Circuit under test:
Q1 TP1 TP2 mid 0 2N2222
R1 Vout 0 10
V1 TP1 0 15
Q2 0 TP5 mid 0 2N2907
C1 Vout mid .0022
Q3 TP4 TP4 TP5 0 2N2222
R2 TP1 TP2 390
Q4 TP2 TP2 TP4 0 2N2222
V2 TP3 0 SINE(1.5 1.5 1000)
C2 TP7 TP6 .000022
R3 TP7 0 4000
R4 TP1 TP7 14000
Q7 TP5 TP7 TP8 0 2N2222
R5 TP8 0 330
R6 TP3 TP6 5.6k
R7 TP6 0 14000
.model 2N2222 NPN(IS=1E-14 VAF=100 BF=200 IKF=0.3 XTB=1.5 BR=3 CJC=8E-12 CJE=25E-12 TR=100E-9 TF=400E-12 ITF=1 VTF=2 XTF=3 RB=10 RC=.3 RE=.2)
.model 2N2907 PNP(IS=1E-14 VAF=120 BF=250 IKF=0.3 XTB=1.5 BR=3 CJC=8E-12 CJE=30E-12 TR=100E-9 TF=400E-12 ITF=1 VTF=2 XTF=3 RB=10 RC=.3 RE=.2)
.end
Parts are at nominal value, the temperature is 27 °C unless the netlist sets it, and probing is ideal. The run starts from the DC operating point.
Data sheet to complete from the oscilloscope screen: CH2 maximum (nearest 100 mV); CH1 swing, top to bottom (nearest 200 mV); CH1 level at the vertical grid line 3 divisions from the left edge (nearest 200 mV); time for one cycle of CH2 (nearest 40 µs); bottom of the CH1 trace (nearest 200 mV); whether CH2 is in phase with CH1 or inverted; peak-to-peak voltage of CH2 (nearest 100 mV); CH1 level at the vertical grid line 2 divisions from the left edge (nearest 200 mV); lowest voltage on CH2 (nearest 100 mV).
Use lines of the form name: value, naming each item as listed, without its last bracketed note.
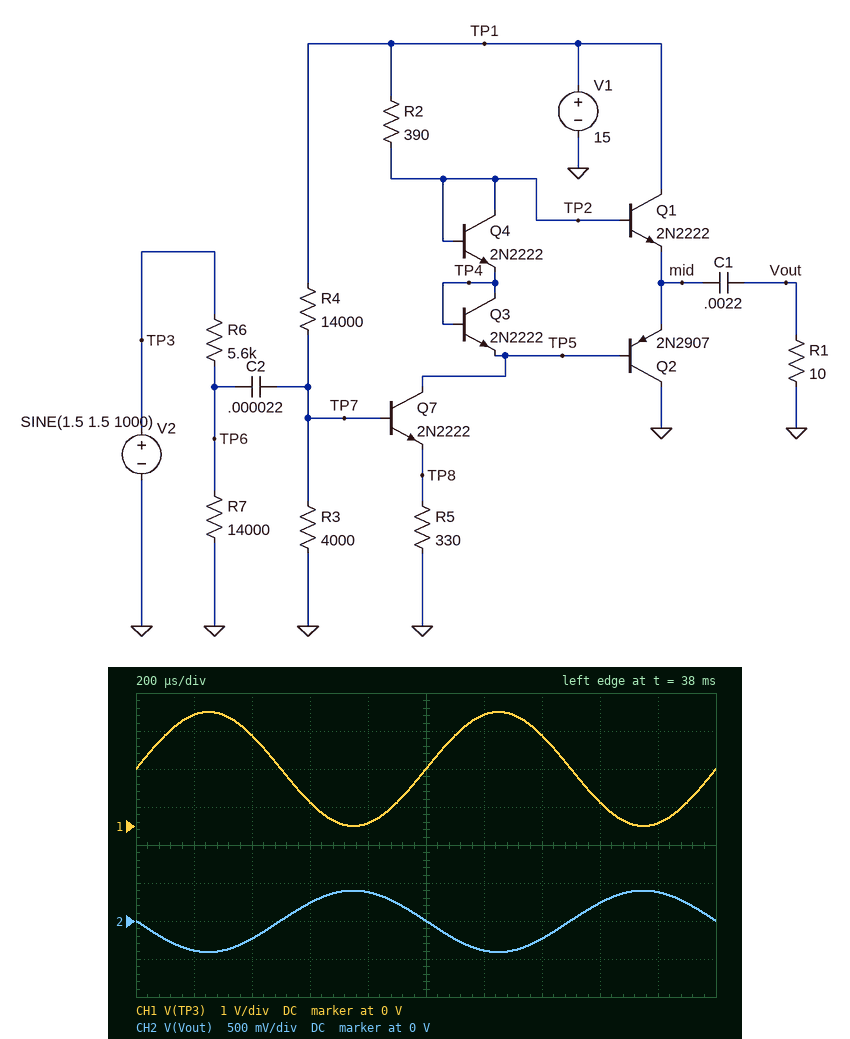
CH2 maximum: 400 mV
CH1 swing, top to bottom: 3.0 V
CH1 level at the vertical grid line 3 divisions from the left edge: 600 mV
time for one cycle of CH2: 1.00 ms
bottom of the CH1 trace: 0 V
whether CH2 is in phase with CH1 or inverted: inverted
peak-to-peak voltage of CH2: 800 mV
CH1 level at the vertical grid line 2 divisions from the left edge: 2.4 V
lowest voltage on CH2: -400 mV
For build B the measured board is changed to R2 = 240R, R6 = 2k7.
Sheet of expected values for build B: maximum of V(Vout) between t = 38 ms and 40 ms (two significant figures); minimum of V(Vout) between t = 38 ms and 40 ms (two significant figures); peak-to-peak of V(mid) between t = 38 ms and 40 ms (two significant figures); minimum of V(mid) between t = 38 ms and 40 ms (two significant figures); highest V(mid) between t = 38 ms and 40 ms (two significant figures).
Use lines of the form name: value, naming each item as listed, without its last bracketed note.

maximum of V(Vout) between t = 38 ms and 40 ms: 410 mV
minimum of V(Vout) between t = 38 ms and 40 ms: -420 mV
peak-to-peak of V(mid) between t = 38 ms and 40 ms: 830 mV
minimum of V(mid) between t = 38 ms and 40 ms: 12 V
highest V(mid) between t = 38 ms and 40 ms: 13 V
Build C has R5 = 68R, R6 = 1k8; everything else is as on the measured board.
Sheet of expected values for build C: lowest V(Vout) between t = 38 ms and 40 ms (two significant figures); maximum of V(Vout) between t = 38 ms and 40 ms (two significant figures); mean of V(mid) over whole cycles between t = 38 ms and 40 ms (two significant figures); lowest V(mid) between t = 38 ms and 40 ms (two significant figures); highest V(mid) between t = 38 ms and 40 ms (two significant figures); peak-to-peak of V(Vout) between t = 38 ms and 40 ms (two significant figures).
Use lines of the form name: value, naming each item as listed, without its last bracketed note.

lowest V(Vout) between t = 38 ms and 40 ms: -1.0 V
maximum of V(Vout) between t = 38 ms and 40 ms: 2.8 V
mean of V(mid) over whole cycles between t = 38 ms and 40 ms: 4.3 V
lowest V(mid) between t = 38 ms and 40 ms: 3.0 V
highest V(mid) between t = 38 ms and 40 ms: 6.7 V
peak-to-peak of V(Vout) between t = 38 ms and 40 ms: 3.8 V
